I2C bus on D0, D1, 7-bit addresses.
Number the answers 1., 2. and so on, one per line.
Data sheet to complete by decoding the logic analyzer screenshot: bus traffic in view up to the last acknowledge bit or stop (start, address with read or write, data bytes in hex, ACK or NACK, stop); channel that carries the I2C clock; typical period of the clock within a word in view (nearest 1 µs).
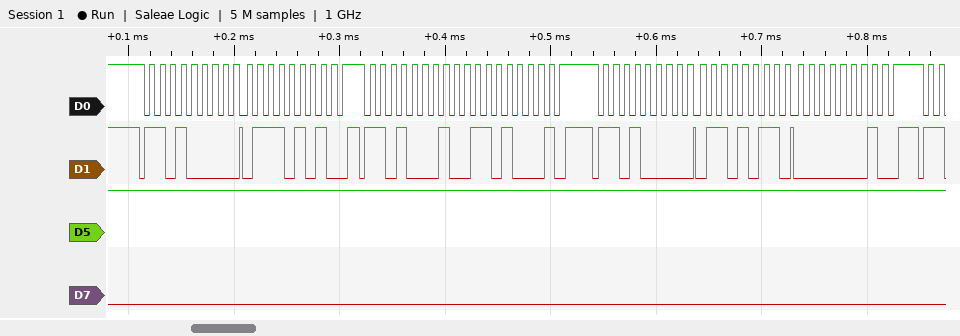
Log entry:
1. start, address 68 write ACK, 75 ACK, stop, start, address 68 read ACK, 68 NACK, stop, start, address 68 write ACK, 6B ACK, 01 ACK, stop
2. D0
3. 10 µs
